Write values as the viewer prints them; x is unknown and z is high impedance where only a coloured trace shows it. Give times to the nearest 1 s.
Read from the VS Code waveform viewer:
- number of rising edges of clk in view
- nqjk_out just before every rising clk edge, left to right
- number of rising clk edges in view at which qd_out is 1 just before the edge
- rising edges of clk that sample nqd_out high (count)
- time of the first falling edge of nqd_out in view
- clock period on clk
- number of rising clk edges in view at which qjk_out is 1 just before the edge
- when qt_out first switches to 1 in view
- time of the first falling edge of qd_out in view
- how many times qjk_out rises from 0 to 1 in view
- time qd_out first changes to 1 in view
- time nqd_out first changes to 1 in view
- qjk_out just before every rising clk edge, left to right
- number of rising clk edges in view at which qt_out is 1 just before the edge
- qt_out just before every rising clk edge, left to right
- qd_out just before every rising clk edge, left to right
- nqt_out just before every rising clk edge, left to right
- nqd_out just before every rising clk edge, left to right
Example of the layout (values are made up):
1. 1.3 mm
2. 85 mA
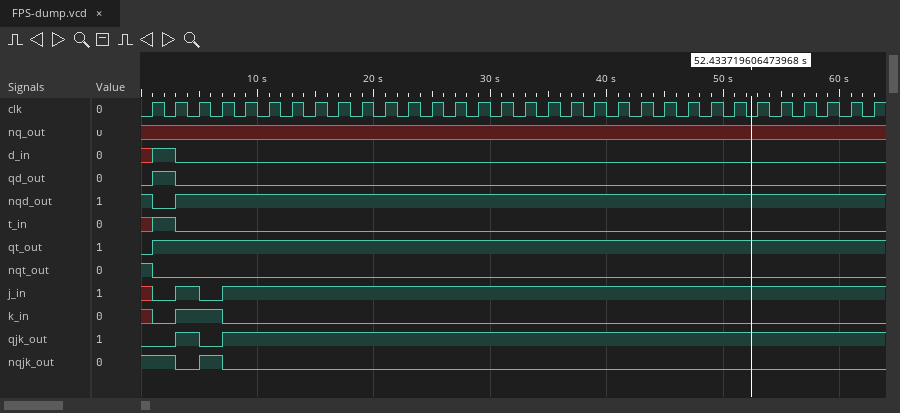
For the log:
1. 32
2. 1 1 0 1 0 0 0 0 0 0 0 0 0 0 0 0 0 0 0 0 0 0 0 0 0 0 0 0 0 0 0 0
3. 1
4. 31
5. 1 s
6. 2 s
7. 29
8. 1 s
9. 3 s
10. 2
11. 1 s
12. 3 s
13. 0 0 1 0 1 1 1 1 1 1 1 1 1 1 1 1 1 1 1 1 1 1 1 1 1 1 1 1 1 1 1 1
14. 31
15. 0 1 1 1 1 1 1 1 1 1 1 1 1 1 1 1 1 1 1 1 1 1 1 1 1 1 1 1 1 1 1 1
16. 0 1 0 0 0 0 0 0 0 0 0 0 0 0 0 0 0 0 0 0 0 0 0 0 0 0 0 0 0 0 0 0
17. 1 0 0 0 0 0 0 0 0 0 0 0 0 0 0 0 0 0 0 0 0 0 0 0 0 0 0 0 0 0 0 0
18. 1 0 1 1 1 1 1 1 1 1 1 1 1 1 1 1 1 1 1 1 1 1 1 1 1 1 1 1 1 1 1 1
